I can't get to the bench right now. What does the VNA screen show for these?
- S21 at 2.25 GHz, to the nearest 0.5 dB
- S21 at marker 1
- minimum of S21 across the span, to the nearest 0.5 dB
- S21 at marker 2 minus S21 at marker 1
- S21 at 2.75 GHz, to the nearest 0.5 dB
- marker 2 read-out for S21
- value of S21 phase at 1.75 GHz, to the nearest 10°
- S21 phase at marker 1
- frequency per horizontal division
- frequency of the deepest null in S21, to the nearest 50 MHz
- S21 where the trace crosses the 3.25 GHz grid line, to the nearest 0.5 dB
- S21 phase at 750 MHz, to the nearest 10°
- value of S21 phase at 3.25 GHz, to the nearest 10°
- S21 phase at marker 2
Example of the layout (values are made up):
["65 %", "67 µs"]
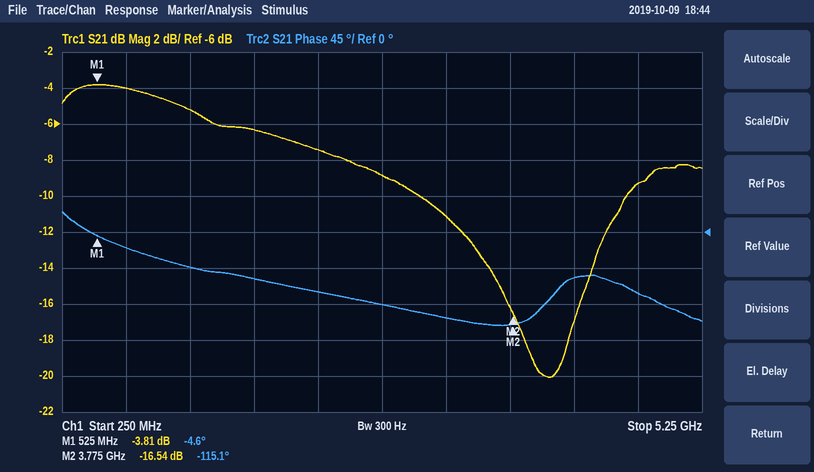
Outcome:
["-7.5 dB", "-3.81 dB", "-20.0 dB", "-12.73 dB", "-9.0 dB", "-16.54 dB", "-60°", "-4.6°", "500 MHz", "4.05 GHz", "-11.0 dB", "-20°", "-110°", "-115.1°"]
